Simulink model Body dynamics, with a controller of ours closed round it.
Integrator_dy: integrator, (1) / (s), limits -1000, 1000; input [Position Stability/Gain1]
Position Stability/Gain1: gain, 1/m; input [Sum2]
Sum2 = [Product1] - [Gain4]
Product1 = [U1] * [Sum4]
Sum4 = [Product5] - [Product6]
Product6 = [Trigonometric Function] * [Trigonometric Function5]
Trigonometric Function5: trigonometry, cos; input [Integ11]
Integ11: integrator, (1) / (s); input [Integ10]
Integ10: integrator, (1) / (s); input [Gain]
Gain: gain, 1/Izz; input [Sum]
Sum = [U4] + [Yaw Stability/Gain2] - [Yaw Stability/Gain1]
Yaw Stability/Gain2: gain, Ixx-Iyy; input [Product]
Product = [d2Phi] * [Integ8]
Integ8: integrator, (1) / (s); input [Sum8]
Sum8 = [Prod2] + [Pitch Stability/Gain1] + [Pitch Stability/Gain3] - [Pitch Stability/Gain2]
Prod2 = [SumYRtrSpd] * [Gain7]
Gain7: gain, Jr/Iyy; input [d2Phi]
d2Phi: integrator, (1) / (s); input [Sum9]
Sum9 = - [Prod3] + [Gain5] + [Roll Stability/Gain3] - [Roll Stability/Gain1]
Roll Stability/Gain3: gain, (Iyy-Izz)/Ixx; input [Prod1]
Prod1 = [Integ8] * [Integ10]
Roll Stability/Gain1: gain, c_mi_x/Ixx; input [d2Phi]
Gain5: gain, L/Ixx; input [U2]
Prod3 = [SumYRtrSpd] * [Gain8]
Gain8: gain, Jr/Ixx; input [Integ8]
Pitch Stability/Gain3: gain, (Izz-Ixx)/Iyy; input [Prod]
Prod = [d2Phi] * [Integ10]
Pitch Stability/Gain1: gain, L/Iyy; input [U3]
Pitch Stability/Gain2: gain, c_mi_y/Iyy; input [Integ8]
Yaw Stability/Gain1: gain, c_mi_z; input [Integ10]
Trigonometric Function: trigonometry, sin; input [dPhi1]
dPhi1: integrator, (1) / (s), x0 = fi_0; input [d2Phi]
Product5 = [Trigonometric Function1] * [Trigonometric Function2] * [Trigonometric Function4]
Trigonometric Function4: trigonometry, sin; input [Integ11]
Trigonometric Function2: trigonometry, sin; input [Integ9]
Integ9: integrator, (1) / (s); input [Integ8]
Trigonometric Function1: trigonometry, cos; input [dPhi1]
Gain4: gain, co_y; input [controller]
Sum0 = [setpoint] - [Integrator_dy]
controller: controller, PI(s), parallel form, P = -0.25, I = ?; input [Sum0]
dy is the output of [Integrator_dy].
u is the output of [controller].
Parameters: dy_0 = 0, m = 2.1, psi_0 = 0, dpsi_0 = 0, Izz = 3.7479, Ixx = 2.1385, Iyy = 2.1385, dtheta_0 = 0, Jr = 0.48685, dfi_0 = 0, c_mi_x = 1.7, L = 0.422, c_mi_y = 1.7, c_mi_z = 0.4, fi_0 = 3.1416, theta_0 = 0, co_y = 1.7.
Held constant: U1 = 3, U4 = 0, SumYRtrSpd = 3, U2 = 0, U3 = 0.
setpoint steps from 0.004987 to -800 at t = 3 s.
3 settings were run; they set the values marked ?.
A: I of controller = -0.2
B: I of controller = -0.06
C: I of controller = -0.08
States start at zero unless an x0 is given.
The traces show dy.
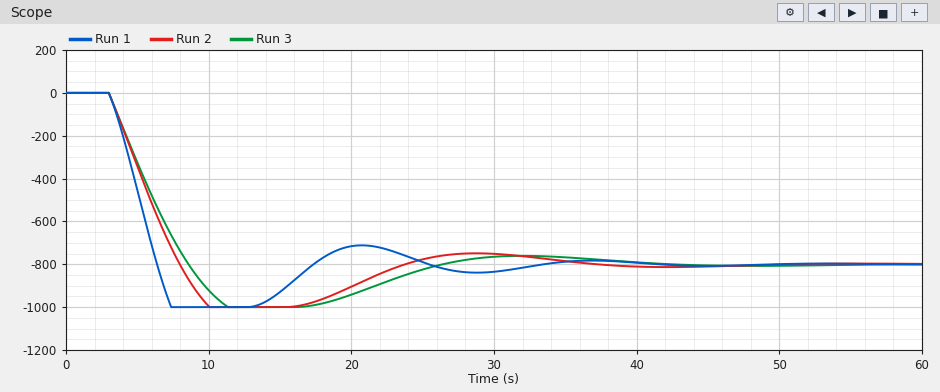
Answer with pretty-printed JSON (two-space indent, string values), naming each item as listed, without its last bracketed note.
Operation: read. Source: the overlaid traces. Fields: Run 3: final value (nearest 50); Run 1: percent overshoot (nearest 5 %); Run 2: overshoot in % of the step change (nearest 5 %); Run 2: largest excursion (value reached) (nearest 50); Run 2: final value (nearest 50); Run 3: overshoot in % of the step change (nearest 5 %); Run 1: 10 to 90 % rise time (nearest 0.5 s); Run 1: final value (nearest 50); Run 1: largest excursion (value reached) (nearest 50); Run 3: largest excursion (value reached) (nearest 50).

{
  "Run 3: final value": "-800",
  "Run 1: percent overshoot": "25 %",
  "Run 2: overshoot in % of the step change": "25 %",
  "Run 2: largest excursion (value reached)": "-1000",
  "Run 2: final value": "-800",
  "Run 3: overshoot in % of the step change": "25 %",
  "Run 1: 10 to 90 % rise time": "2.5 s",
  "Run 1: final value": "-800",
  "Run 1: largest excursion (value reached)": "-1000",
  "Run 3: largest excursion (value reached)": "-1000"
}
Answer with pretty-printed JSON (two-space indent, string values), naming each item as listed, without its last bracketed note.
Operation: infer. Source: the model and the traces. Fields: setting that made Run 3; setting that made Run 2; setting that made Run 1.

{
  "setting that made Run 3": "B",
  "setting that made Run 2": "C",
  "setting that made Run 1": "A"
}
